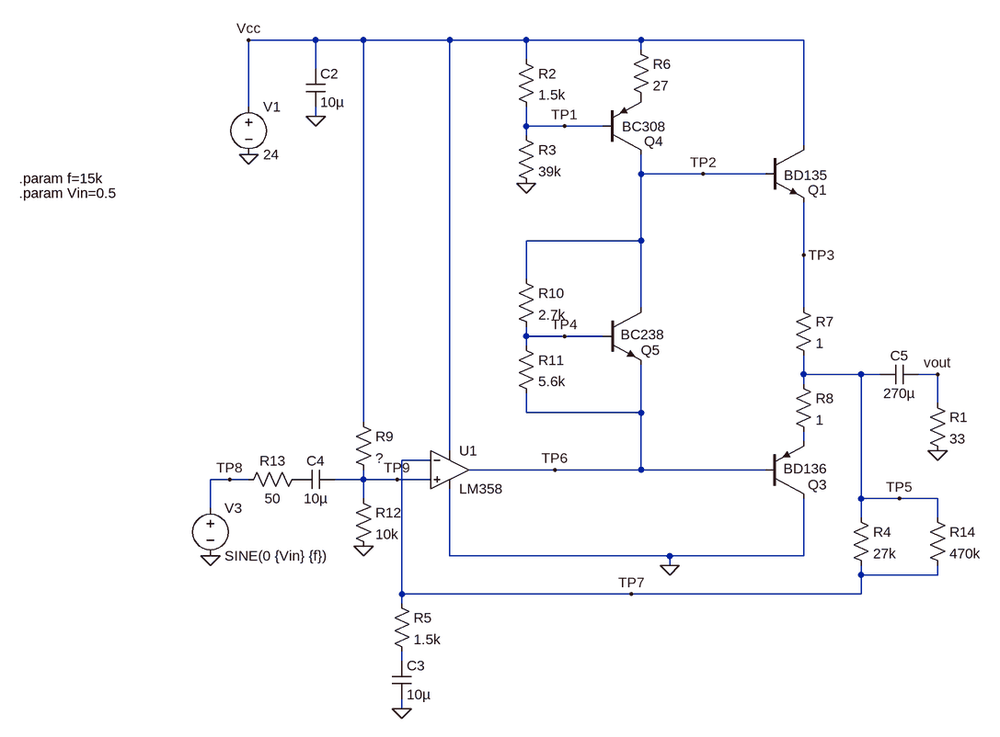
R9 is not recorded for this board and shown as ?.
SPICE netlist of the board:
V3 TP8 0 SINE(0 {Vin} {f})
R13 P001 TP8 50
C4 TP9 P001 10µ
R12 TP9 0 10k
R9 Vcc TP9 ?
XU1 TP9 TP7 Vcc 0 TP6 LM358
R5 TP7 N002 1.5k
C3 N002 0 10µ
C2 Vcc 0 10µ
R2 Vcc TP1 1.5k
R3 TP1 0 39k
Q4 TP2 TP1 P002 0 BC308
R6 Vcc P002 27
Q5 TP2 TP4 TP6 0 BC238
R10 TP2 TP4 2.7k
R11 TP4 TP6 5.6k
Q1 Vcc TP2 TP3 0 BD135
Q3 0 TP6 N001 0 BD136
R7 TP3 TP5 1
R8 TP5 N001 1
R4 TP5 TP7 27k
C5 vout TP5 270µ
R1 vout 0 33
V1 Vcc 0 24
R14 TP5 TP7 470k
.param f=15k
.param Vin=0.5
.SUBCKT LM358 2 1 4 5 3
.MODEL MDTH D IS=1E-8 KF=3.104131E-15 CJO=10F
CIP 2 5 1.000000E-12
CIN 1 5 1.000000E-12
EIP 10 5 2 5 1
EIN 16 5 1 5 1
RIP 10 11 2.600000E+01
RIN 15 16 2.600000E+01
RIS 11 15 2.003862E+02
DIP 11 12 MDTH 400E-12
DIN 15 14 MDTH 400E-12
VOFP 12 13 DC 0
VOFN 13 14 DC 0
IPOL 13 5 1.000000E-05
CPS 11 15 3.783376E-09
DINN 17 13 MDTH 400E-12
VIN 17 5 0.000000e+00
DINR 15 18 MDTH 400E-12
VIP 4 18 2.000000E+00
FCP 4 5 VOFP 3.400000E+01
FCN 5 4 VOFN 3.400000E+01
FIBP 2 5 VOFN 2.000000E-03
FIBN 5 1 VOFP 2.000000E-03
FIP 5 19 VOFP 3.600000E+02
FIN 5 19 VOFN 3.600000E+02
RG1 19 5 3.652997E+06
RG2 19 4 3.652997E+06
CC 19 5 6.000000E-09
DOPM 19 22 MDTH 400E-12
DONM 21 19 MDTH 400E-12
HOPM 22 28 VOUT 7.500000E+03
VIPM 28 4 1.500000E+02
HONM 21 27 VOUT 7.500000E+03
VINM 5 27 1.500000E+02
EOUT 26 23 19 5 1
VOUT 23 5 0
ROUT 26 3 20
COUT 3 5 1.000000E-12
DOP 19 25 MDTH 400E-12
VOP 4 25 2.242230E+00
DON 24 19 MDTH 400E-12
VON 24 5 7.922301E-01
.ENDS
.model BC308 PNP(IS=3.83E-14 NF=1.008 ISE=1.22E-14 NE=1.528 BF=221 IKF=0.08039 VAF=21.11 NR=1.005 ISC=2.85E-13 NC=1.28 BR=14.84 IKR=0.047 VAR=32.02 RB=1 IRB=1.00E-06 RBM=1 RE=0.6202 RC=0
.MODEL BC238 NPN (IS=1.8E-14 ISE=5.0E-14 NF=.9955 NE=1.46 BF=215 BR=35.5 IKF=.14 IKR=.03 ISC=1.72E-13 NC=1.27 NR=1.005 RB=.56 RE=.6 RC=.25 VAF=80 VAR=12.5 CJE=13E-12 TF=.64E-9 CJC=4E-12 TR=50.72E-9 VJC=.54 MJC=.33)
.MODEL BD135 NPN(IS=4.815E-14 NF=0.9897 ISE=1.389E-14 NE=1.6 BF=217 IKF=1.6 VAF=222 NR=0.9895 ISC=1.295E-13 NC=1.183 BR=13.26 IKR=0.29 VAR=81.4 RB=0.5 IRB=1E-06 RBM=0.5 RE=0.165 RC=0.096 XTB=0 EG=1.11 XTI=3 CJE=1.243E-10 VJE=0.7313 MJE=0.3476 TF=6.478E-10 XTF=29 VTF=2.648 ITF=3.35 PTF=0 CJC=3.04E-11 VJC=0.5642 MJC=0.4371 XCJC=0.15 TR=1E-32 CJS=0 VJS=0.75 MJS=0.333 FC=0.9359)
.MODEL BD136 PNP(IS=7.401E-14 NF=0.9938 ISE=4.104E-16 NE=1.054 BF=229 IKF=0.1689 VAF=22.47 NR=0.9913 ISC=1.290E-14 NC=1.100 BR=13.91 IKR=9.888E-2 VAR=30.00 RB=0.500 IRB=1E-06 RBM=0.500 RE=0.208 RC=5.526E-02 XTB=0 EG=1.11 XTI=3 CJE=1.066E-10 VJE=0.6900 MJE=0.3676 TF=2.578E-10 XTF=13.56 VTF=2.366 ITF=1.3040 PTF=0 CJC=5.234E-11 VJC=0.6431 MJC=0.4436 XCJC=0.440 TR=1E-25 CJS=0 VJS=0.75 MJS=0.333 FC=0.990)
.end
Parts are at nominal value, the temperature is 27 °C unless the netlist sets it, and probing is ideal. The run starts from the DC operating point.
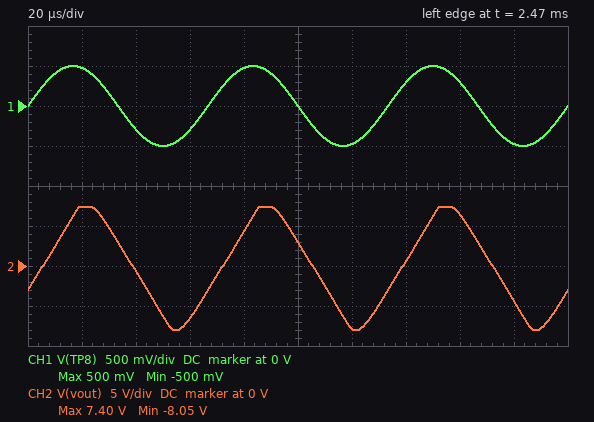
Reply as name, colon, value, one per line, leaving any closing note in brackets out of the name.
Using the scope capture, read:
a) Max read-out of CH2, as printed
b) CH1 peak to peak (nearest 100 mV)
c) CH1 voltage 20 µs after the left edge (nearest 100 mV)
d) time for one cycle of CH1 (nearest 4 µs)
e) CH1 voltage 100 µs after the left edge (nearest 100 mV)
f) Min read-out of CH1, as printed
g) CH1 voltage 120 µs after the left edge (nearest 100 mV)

Max read-out of CH2, as printed: 7.40 V
CH1 peak to peak: 1.0 V
CH1 voltage 20 µs after the left edge: 500 mV
time for one cycle of CH1: 68 µs
CH1 voltage 100 µs after the left edge: 0 V
Min read-out of CH1, as printed: -500 mV
CH1 voltage 120 µs after the left edge: -500 mV
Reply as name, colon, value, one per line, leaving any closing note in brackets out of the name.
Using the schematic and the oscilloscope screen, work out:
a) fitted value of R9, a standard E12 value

fitted value of R9, a standard E12 value: 5.6 kΩ
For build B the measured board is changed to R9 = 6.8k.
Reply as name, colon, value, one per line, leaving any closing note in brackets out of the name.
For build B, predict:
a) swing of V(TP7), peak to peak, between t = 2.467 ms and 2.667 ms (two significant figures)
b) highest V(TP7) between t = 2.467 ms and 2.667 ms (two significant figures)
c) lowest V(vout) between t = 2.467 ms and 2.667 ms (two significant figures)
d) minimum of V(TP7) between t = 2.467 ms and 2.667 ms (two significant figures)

swing of V(TP7), peak to peak, between t = 2.467 ms and 2.667 ms: 890 mV
highest V(TP7) between t = 2.467 ms and 2.667 ms: 15 V
lowest V(vout) between t = 2.467 ms and 2.667 ms: -8.1 V
minimum of V(TP7) between t = 2.467 ms and 2.667 ms: 14 V
